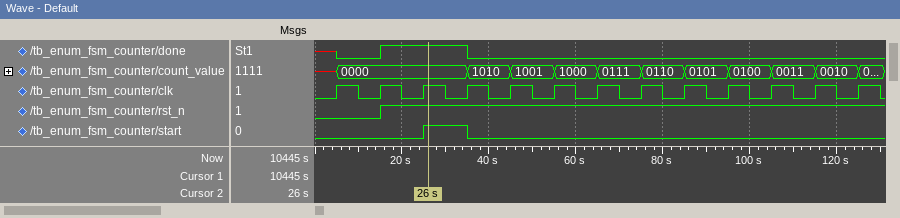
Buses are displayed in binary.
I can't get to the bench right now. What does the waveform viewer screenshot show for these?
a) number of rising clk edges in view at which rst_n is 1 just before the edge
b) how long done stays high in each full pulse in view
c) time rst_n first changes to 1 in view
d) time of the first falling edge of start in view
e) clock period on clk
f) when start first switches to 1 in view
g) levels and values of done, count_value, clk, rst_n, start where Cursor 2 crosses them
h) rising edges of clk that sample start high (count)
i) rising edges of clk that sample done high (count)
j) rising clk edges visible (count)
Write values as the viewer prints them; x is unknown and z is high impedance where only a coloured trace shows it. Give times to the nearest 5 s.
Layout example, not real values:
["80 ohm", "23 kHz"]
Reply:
["11", "20 s", "15 s", "35 s", "10 s", "25 s", "done=1, count_value=0000, clk=1, rst_n=1, start=1", "1", "2", "13"]
